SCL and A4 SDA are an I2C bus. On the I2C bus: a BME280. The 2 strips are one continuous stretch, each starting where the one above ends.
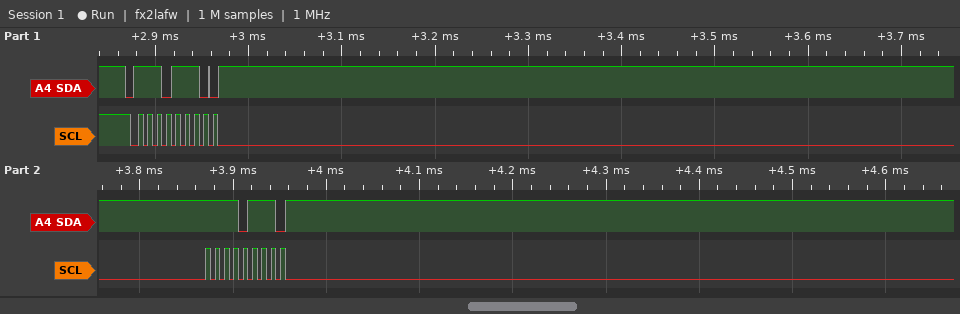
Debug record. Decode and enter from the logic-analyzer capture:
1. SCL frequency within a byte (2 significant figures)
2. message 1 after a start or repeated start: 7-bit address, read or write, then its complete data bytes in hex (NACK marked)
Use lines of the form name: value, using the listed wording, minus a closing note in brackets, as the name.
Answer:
SCL frequency within a byte: 100 kHz
message 1 after a start or repeated start: 7-bit address, read or write, then its complete data bytes in hex: 0x77 write: F7
